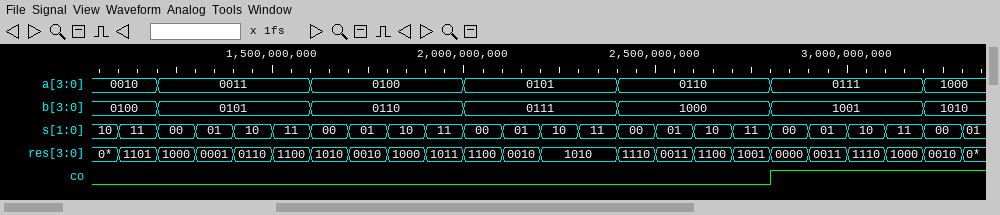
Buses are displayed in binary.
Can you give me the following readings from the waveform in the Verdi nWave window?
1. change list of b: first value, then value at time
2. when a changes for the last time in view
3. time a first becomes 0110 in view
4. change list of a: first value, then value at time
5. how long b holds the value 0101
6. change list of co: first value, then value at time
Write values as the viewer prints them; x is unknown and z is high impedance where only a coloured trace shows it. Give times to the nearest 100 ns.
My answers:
0100, 0101 at 1200 ns, 0110 at 1600 ns, 0111 at 2000 ns, 1000 at 2400 ns, 1001 at 2800 ns, 1010 at 3200 ns
3200 ns
2400 ns
0010, 0011 at 1200 ns, 0100 at 1600 ns, 0101 at 2000 ns, 0110 at 2400 ns, 0111 at 2800 ns, 1000 at 3200 ns
400 ns
0, 1 at 2800 ns
